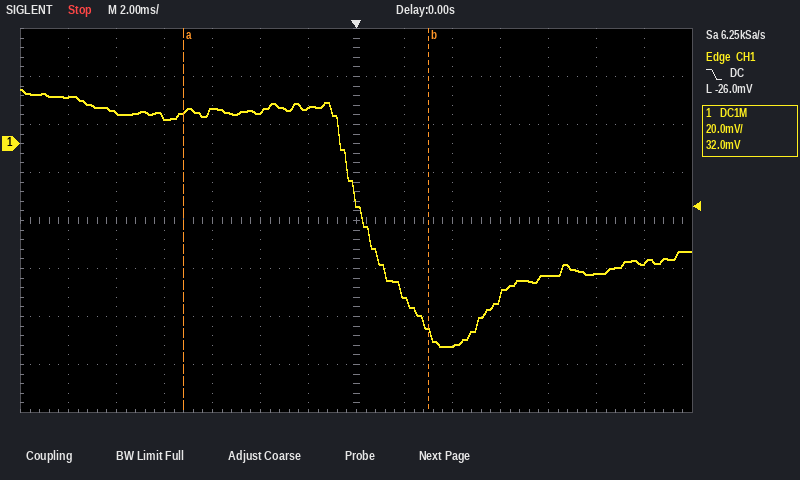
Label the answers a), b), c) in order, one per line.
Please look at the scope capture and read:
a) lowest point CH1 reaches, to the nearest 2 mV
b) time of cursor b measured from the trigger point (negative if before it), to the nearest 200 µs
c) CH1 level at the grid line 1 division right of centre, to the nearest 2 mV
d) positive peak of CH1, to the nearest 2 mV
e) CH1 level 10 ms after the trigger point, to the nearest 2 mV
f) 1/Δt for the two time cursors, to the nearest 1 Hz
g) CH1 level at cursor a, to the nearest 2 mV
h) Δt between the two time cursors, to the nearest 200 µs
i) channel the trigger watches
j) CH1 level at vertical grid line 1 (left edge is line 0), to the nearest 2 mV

a) -84 mV
b) +3.0 ms
c) -64 mV
d) 22 mV
e) -54 mV
f) 98 Hz
g) 14 mV
h) 10.2 ms
i) CH1
j) 20 mV
